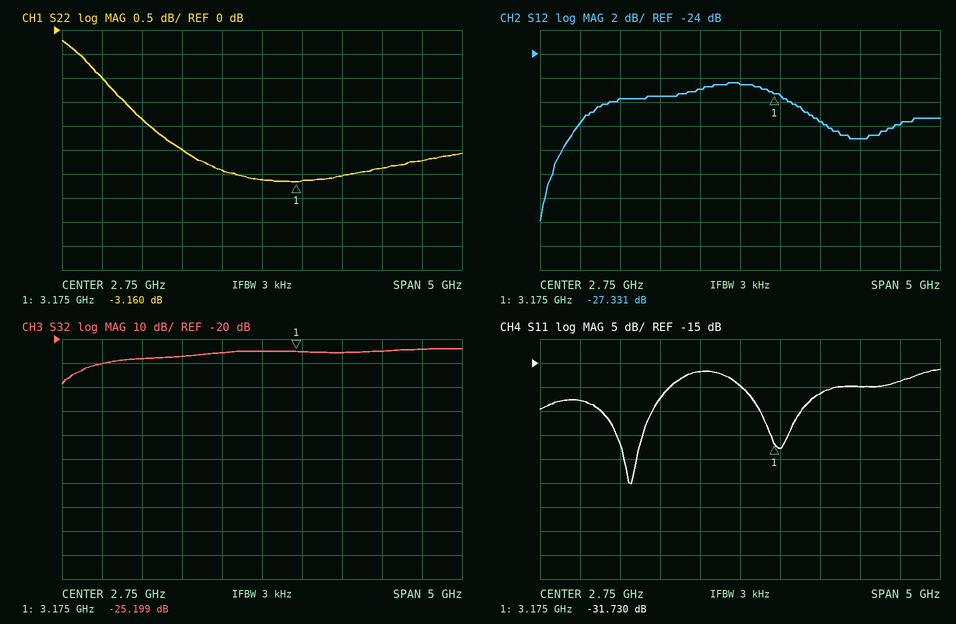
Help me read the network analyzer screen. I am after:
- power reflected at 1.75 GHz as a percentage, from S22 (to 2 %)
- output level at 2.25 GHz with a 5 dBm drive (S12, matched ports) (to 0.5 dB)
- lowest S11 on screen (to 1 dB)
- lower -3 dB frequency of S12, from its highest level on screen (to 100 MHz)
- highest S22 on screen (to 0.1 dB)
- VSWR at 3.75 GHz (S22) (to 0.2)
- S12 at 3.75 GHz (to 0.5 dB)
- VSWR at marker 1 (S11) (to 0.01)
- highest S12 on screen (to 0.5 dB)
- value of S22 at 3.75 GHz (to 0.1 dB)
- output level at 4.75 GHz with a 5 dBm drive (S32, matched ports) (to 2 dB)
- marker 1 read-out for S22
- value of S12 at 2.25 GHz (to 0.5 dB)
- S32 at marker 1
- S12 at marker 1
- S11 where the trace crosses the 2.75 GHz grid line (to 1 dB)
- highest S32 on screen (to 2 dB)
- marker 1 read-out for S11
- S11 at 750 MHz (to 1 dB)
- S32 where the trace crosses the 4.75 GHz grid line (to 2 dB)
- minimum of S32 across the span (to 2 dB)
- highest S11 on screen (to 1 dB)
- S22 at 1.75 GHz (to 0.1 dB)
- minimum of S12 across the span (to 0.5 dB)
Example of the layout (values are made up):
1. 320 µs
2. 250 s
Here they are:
1. 56 %
2. -22.0 dBm
3. -40 dB
4. 800 MHz
5. -0.2 dB
6. 5.8
7. -29.5 dB
8. 1.05
9. -26.5 dB
10. -3.0 dB
11. -20 dBm
12. -3.160 dB
13. -27.0 dB
14. -25.199 dB
15. -27.331 dB
16. -20 dB
17. -24 dB
18. -31.730 dB
19. -23 dB
20. -24 dB
21. -38 dB
22. -16 dB
23. -2.5 dB
24. -38.0 dB
